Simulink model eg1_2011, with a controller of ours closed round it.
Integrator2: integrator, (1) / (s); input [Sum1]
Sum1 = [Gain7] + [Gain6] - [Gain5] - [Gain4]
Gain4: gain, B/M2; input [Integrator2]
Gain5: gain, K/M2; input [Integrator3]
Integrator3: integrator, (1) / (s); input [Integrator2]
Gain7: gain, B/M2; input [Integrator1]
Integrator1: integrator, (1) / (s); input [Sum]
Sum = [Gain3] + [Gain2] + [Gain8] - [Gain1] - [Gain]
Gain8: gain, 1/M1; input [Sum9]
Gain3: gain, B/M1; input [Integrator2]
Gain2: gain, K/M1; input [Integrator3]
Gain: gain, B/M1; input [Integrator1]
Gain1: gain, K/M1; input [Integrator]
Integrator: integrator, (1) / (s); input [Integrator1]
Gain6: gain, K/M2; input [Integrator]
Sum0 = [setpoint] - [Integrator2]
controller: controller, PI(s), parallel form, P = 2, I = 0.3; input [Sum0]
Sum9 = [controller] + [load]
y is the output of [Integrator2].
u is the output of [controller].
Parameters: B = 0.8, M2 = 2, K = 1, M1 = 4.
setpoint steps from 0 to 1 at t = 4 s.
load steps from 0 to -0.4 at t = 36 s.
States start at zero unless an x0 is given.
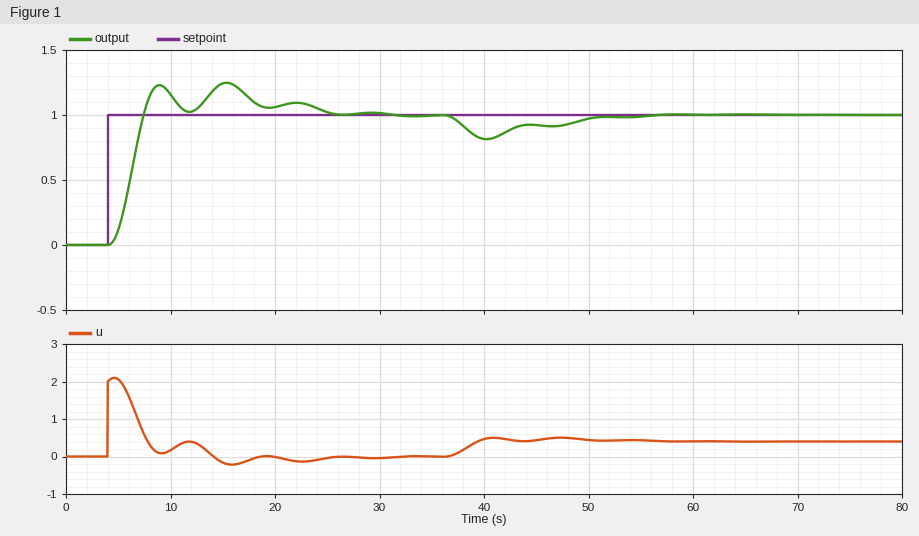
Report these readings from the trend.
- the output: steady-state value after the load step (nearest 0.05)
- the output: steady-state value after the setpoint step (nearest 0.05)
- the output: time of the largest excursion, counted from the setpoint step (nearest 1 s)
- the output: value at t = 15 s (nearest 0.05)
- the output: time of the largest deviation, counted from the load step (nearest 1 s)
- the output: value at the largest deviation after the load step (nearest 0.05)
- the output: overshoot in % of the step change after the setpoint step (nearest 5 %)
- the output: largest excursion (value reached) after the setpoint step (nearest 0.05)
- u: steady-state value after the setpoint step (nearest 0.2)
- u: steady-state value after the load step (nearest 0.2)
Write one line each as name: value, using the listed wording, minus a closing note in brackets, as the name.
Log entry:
the output: steady-state value after the load step: 1.00
the output: steady-state value after the setpoint step: 1.00
the output: time of the largest excursion, counted from the setpoint step: 11 s
the output: value at t = 15 s: 1.25
the output: time of the largest deviation, counted from the load step: 4 s
the output: value at the largest deviation after the load step: 0.80
the output: overshoot in % of the step change after the setpoint step: 25 %
the output: largest excursion (value reached) after the setpoint step: 1.25
u: steady-state value after the setpoint step: 0.0
u: steady-state value after the load step: 0.4
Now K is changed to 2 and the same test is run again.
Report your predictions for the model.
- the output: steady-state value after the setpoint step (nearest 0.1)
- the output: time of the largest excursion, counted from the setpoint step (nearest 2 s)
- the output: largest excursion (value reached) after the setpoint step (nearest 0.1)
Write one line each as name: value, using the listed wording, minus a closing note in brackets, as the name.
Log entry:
the output: steady-state value after the setpoint step: 1.0
the output: time of the largest excursion, counted from the setpoint step: 8 s
the output: largest excursion (value reached) after the setpoint step: 1.3
